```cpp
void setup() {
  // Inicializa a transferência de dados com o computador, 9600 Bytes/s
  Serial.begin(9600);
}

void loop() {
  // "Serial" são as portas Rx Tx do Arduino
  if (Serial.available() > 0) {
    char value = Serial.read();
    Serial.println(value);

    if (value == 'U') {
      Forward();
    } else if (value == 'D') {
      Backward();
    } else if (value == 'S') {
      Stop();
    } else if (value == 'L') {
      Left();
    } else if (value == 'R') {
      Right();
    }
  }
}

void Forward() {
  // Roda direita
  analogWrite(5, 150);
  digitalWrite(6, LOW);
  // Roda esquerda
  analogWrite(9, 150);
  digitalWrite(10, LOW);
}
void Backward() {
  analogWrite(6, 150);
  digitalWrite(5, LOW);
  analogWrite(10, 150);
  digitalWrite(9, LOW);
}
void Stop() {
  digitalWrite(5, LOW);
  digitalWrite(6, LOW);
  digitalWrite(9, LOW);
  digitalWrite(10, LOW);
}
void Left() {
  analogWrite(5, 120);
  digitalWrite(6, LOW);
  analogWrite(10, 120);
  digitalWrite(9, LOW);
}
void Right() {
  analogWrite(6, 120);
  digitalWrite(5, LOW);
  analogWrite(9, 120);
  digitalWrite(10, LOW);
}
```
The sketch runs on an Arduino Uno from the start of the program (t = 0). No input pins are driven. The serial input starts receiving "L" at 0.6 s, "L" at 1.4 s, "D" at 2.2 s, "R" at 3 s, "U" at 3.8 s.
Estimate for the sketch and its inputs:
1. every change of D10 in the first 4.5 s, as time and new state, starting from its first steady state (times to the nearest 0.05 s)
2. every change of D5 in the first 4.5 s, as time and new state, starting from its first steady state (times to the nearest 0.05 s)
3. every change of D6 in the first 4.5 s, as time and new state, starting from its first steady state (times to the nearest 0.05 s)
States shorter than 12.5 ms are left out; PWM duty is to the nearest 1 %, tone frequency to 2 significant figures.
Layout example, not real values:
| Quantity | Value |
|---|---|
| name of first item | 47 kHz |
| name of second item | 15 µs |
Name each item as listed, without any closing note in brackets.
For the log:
| Quantity | Value |
|---|---|
| every change of D10 in the first 4.5 s, as time and new state, starting from its first steady state | 0.6 s PWM 47 %; 2.2 s PWM 59 %; 3 s low |
| every change of D5 in the first 4.5 s, as time and new state, starting from its first steady state | 0.6 s PWM 47 %; 2.2 s low; 3.8 s PWM 59 % |
| every change of D6 in the first 4.5 s, as time and new state, starting from its first steady state | 2.2 s PWM 59 %; 3 s PWM 47 %; 3.8 s low |
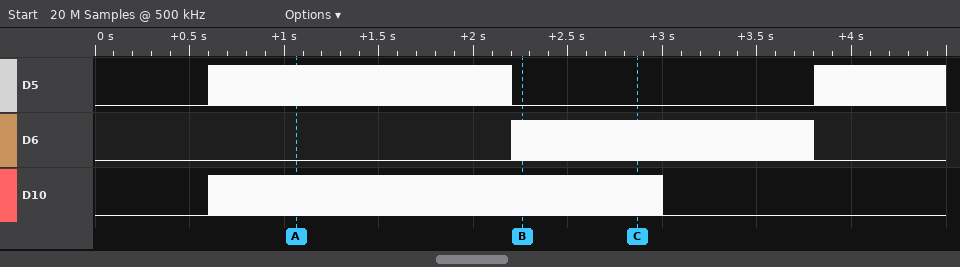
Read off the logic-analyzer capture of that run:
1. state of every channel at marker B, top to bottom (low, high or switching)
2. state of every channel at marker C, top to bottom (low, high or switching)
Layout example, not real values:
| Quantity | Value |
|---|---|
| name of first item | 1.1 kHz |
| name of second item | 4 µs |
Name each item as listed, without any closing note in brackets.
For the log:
| Quantity | Value |
|---|---|
| state of every channel at marker B, top to bottom | D5 low, D6 switching, D10 switching |
| state of every channel at marker C, top to bottom | D5 low, D6 switching, D10 switching |
